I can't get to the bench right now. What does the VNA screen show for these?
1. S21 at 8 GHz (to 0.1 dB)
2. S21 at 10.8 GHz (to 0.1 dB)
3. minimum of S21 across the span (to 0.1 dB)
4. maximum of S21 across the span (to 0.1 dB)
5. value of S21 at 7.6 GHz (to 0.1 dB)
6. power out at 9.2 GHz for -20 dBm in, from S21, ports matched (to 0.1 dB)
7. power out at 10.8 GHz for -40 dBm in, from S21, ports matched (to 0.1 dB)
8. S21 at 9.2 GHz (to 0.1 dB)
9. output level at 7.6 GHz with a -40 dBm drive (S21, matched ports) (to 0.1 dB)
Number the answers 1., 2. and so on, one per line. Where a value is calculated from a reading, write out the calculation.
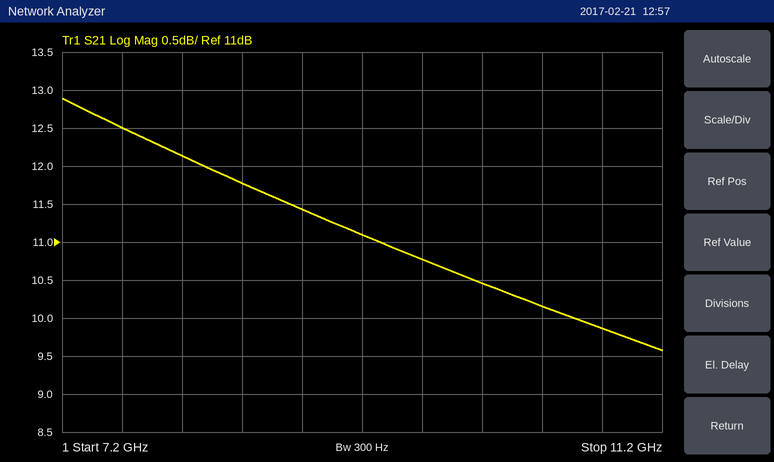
1. 12.1 dB
2. 9.9 dB
3. 9.6 dB
4. 12.9 dB
5. 12.5 dB
6. -20 dBm + (11.1 dB) = -8.9 dBm
7. -40 dBm + (9.9 dB) = -30.1 dBm
8. 11.1 dB
9. -40 dBm + (12.5 dB) = -27.5 dBm
